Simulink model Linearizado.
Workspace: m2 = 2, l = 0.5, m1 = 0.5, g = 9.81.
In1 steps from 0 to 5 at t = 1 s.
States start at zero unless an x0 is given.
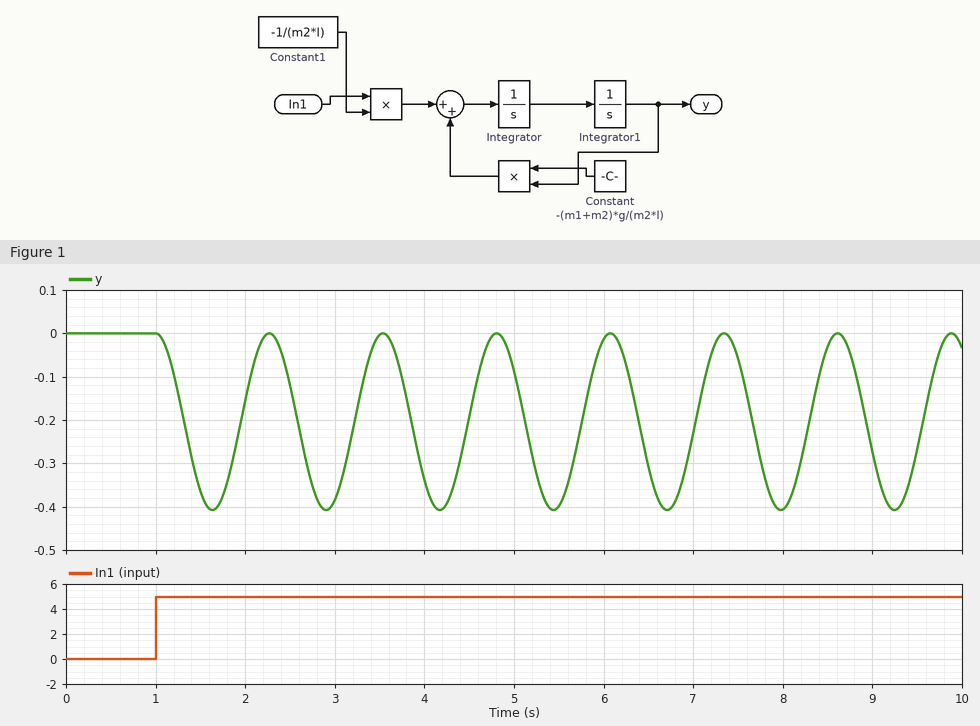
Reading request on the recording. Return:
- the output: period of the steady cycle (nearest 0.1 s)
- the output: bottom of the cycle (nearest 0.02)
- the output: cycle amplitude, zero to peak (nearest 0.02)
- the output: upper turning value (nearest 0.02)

1.3 s
-0.40
0.20
0.00
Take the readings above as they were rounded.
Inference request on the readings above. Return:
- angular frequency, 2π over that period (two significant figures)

4.8 rad/s
